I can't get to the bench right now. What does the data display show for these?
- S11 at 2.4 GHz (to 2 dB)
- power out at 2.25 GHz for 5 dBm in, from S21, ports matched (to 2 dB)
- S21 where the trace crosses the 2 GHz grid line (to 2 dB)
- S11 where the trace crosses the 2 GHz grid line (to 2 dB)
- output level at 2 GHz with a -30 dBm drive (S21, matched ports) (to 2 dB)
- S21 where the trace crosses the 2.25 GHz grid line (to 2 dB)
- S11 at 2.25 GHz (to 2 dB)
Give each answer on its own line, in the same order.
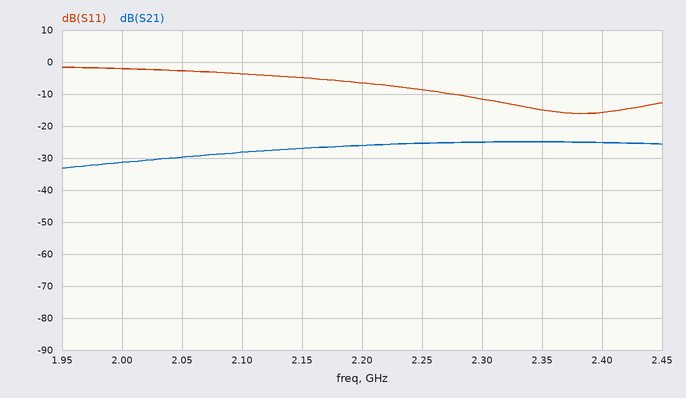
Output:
-16 dB
-20 dBm
-32 dB
-2 dB
-62 dBm
-26 dB
-8 dB
